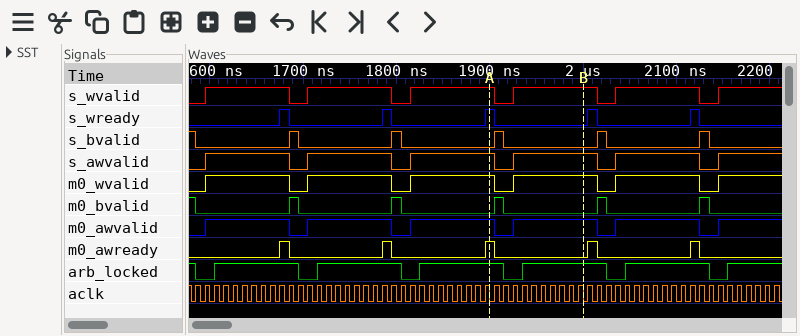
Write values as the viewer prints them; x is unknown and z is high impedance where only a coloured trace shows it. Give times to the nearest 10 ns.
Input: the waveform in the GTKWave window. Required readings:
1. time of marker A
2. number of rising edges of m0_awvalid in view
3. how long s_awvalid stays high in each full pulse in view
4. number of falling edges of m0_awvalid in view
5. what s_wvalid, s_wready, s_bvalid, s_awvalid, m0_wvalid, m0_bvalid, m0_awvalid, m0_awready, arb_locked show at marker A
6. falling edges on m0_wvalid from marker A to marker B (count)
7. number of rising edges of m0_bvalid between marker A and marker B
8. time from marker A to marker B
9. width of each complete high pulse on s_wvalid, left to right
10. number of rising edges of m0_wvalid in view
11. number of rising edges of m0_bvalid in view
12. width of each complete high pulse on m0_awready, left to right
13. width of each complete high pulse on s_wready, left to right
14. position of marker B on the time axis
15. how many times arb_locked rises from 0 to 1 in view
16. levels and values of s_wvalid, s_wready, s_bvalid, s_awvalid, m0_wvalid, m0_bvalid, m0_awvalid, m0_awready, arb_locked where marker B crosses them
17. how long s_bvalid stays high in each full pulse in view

1900 ns
6
90 ns, 90 ns, 90 ns, 90 ns, 90 ns
5
s_wvalid=1, s_wready=1, s_bvalid=0, s_awvalid=1, m0_wvalid=1, m0_bvalid=0, m0_awvalid=1, m0_awready=1, arb_locked=1
1
1
100 ns
90 ns, 90 ns, 90 ns, 90 ns, 90 ns
6
5
10 ns, 10 ns, 10 ns, 10 ns, 10 ns
10 ns, 10 ns, 10 ns, 10 ns, 10 ns
2000 ns
6
s_wvalid=1, s_wready=0, s_bvalid=0, s_awvalid=1, m0_wvalid=1, m0_bvalid=0, m0_awvalid=1, m0_awready=0, arb_locked=1
10 ns, 10 ns, 10 ns, 10 ns, 10 ns
